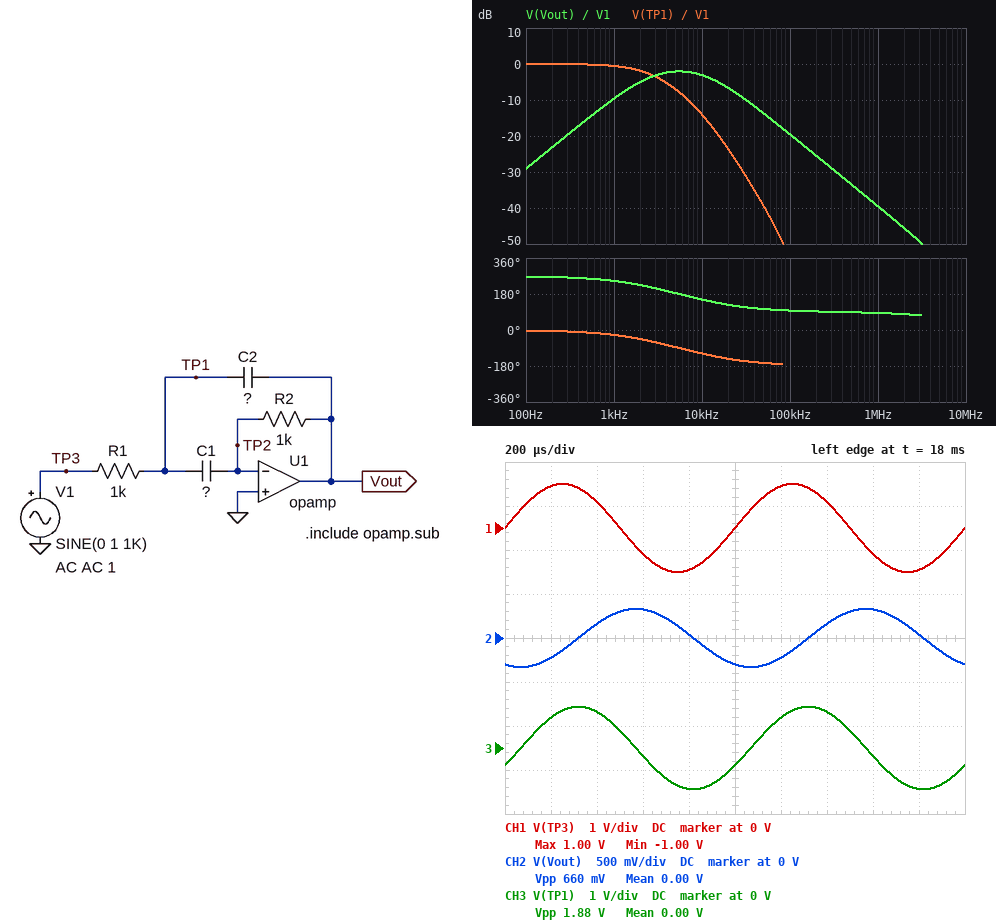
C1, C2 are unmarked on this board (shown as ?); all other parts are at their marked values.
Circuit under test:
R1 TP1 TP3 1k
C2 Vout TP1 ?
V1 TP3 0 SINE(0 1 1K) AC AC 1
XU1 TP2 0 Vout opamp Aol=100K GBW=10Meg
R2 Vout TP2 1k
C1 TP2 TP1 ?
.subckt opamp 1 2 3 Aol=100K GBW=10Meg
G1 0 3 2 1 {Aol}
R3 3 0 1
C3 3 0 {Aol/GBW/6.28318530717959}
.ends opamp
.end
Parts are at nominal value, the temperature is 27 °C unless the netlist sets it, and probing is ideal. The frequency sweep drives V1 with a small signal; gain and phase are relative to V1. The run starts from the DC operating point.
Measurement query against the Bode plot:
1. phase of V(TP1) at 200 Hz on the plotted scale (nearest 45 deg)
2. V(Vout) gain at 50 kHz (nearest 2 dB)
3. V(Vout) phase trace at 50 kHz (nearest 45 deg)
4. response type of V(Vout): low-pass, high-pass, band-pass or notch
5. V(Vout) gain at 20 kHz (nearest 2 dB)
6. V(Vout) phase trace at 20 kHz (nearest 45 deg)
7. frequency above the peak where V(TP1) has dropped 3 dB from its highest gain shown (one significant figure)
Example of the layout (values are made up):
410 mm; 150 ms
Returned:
0 deg; -14 dB; 90 deg; band-pass; -6 dB; 135 deg; 3 kHz
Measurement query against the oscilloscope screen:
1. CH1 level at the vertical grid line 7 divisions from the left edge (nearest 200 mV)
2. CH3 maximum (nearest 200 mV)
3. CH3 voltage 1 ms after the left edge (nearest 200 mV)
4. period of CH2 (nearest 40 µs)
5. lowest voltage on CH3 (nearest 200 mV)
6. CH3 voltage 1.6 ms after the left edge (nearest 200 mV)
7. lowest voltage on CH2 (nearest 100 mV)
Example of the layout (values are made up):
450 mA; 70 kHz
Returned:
600 mV; 1.0 V; -400 mV; 1.00 ms; -1.0 V; -200 mV; -300 mV
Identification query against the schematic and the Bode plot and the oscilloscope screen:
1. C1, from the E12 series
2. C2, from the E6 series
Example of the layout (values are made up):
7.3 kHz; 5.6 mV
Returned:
56 nF; 15 nF
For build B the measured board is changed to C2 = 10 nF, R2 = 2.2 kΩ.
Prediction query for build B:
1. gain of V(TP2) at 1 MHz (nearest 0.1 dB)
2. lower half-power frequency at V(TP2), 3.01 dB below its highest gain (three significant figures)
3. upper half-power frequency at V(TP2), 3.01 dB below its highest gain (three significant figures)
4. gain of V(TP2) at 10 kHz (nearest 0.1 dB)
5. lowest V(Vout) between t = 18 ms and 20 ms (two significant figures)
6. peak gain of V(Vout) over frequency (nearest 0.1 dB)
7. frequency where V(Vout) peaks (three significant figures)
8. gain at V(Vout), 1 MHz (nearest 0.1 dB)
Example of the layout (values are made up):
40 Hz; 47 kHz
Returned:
-56.0 dB; 6.44 kHz; 10.0 MHz; -57.3 dB; -750 mV; 5.4 dB; 4.53 kHz; -36.0 dB
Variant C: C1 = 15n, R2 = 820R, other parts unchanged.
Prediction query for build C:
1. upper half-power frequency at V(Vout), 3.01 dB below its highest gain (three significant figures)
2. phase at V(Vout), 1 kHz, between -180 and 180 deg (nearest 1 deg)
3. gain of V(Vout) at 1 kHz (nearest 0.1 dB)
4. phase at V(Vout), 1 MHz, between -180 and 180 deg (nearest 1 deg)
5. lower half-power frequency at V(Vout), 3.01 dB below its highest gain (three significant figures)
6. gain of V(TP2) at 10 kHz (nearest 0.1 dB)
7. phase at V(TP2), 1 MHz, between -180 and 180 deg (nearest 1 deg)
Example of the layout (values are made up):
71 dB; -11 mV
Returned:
30.4 kHz; -101 deg; -22.3 dB; 86 deg; 4.52 kHz; -67.8 dB; -4 deg
